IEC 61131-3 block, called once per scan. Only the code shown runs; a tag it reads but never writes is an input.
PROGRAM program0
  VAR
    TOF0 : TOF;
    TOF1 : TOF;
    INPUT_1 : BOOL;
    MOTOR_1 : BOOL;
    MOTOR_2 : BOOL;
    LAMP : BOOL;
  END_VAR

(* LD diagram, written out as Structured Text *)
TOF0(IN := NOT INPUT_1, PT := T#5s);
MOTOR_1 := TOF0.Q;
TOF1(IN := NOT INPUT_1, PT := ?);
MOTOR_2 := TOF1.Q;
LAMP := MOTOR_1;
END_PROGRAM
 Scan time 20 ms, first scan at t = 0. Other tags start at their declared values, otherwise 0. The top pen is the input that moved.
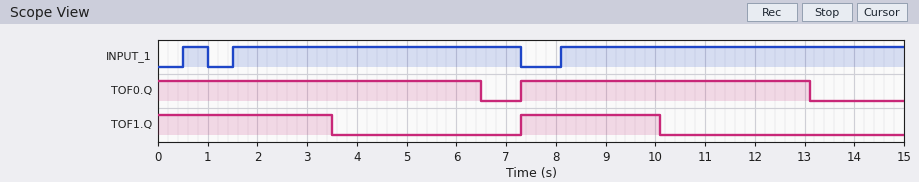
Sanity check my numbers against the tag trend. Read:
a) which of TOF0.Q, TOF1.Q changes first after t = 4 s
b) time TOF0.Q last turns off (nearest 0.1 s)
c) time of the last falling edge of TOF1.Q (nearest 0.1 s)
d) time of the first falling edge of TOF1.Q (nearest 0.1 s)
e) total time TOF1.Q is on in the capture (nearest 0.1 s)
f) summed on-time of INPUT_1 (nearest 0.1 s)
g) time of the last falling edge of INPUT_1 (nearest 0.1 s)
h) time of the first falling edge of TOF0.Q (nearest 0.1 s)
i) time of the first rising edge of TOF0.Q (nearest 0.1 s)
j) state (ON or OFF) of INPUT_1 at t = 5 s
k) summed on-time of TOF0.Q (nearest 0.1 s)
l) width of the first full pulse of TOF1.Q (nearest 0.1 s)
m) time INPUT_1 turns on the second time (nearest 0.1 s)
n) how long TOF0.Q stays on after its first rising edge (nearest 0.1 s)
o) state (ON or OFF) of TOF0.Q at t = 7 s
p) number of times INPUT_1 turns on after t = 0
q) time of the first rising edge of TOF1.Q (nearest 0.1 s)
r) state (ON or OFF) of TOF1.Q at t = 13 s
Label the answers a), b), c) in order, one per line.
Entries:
a) TOF0.Q
b) 13.1 s
c) 10.1 s
d) 3.5 s
e) 6.3 s
f) 13.2 s
g) 7.3 s
h) 6.5 s
i) 7.3 s
j) ON
k) 12.3 s
l) 2.8 s
m) 1.5 s
n) 5.8 s
o) OFF
p) 3
q) 7.3 s
r) OFF
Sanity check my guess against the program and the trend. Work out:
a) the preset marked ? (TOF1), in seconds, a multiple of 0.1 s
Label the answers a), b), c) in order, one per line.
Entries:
a) 2.0 s
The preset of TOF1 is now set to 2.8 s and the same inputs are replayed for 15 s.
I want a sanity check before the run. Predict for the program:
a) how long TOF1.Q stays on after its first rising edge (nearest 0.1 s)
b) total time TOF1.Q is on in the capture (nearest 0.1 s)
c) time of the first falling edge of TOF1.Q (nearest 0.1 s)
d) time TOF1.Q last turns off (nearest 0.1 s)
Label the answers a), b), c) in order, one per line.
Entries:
a) 3.6 s
b) 7.9 s
c) 4.3 s
d) 10.9 s
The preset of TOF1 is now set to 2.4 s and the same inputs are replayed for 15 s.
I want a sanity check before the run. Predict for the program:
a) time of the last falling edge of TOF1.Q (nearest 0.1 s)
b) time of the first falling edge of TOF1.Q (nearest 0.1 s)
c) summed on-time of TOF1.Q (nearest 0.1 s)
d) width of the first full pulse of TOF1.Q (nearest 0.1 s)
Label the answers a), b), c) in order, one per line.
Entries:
a) 10.5 s
b) 3.9 s
c) 7.1 s
d) 3.2 s
